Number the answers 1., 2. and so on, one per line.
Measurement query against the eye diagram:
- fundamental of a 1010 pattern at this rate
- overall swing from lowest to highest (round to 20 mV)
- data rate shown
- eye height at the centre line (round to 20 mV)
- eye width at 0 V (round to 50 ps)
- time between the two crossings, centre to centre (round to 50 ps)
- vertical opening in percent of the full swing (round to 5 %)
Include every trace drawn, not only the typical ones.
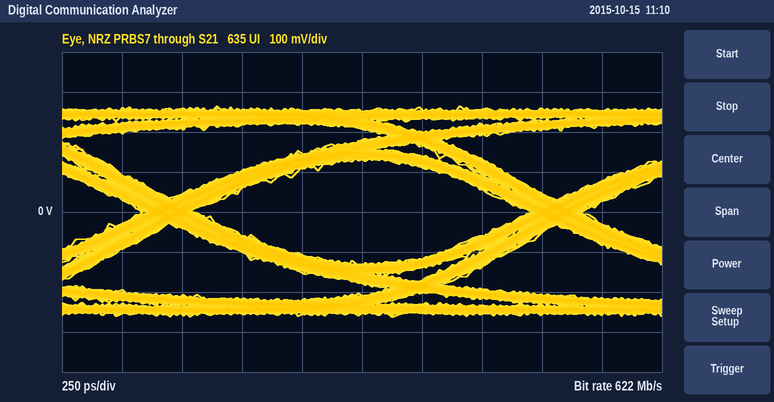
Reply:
1. 311 MHz
2. 520 mV
3. 622 Mb/s
4. 260 mV
5. 1.40 ns
6. 1.60 ns
7. 50 %
